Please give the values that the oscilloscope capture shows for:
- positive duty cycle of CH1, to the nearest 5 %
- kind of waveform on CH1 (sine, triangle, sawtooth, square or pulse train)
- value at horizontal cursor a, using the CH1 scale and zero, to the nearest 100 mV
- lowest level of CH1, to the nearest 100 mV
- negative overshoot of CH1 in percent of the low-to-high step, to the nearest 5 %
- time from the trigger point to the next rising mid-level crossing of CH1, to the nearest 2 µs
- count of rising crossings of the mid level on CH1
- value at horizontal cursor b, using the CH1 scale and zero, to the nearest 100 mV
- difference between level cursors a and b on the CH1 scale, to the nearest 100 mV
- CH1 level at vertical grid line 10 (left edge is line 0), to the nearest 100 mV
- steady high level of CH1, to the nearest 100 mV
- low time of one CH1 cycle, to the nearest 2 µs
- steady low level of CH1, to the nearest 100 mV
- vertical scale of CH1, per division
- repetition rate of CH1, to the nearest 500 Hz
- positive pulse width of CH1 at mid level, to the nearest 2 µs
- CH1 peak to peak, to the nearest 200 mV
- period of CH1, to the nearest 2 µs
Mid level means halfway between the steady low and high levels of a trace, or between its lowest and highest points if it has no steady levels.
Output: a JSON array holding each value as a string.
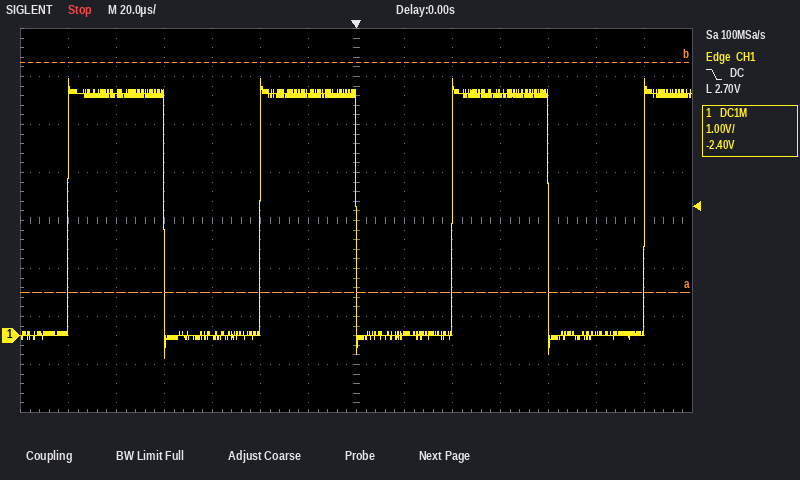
["50 %", "square", "900 mV", "-500 mV", "10 %", "40 µs", "4", "5.7 V", "4.8 V", "5.0 V", "5.0 V", "40 µs", "0.0 V", "1 V", "12.5 kHz", "40 µs", "5.8 V", "80 µs"]
